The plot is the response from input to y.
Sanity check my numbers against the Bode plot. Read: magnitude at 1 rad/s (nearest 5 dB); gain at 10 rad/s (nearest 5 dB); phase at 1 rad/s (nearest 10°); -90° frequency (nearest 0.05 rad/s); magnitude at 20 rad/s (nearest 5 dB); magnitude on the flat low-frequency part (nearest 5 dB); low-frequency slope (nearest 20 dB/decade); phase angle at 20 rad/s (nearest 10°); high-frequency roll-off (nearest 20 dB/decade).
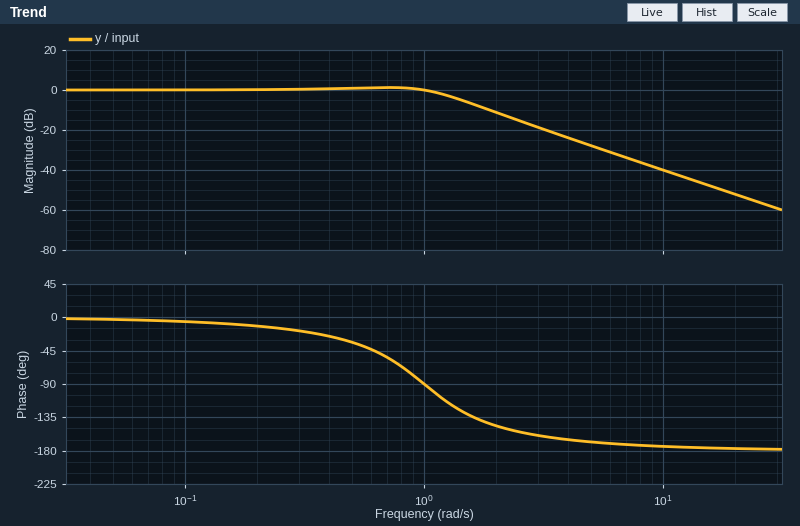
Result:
0 dB
-40 dB
-90°
1.00 rad/s
-50 dB
0 dB
0 dB/decade
-180°
-40 dB/decade
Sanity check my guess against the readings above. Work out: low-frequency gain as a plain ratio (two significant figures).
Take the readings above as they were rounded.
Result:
1.0
